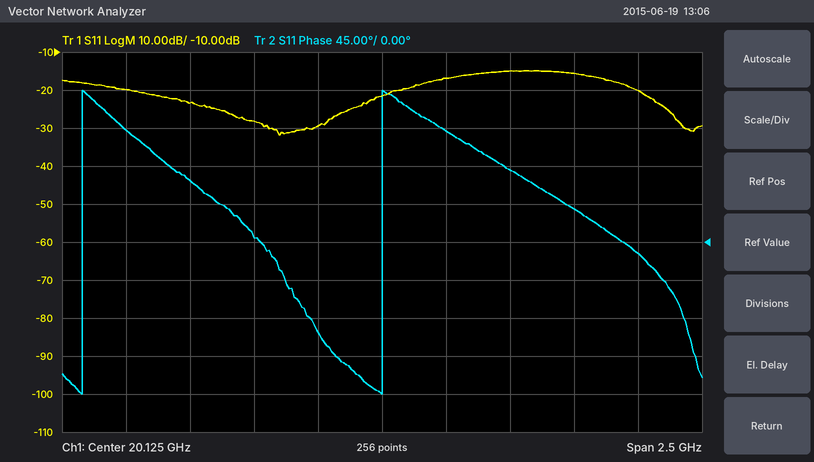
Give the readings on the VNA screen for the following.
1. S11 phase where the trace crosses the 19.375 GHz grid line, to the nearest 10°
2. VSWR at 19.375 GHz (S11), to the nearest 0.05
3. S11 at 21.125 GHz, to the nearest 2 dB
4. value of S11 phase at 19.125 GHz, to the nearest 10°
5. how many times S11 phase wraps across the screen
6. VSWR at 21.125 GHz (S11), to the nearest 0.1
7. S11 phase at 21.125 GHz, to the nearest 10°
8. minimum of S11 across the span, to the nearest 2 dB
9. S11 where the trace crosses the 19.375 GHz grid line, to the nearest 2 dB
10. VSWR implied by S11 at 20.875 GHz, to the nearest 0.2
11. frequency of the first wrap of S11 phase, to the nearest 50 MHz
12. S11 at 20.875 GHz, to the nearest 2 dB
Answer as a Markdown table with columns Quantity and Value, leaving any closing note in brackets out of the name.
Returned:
| Quantity | Value |
|---|---|
| S11 phase where the trace crosses the 19.375 GHz grid line, to the nearest 10° | 70° |
| VSWR at 19.375 GHz (S11), to the nearest 0.05 | 1.15 |
| S11 at 21.125 GHz, to the nearest 2 dB | -20 dB |
| value of S11 phase at 19.125 GHz, to the nearest 10° | 130° |
| how many times S11 phase wraps across the screen | 2 |
| VSWR at 21.125 GHz (S11), to the nearest 0.1 | 1.2 |
| S11 phase at 21.125 GHz, to the nearest 10° | -10° |
| minimum of S11 across the span, to the nearest 2 dB | -32 dB |
| S11 where the trace crosses the 19.375 GHz grid line, to the nearest 2 dB | -24 dB |
| VSWR implied by S11 at 20.875 GHz, to the nearest 0.2 | 1.4 |
| frequency of the first wrap of S11 phase, to the nearest 50 MHz | 18.95 GHz |
| S11 at 20.875 GHz, to the nearest 2 dB | -16 dB |
